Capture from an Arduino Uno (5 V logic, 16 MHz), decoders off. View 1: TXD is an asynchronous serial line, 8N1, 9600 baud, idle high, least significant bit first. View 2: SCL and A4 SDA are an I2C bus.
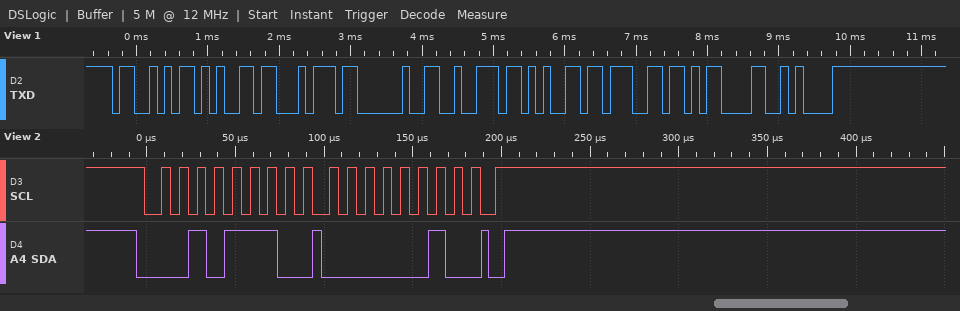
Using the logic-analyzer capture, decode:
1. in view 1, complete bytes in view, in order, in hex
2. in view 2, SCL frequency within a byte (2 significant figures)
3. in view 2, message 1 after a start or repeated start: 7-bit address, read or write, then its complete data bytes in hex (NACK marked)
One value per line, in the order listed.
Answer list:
53 65 74 20 72 65 67 0D 0A
100 kHz
0x17 write: 02
